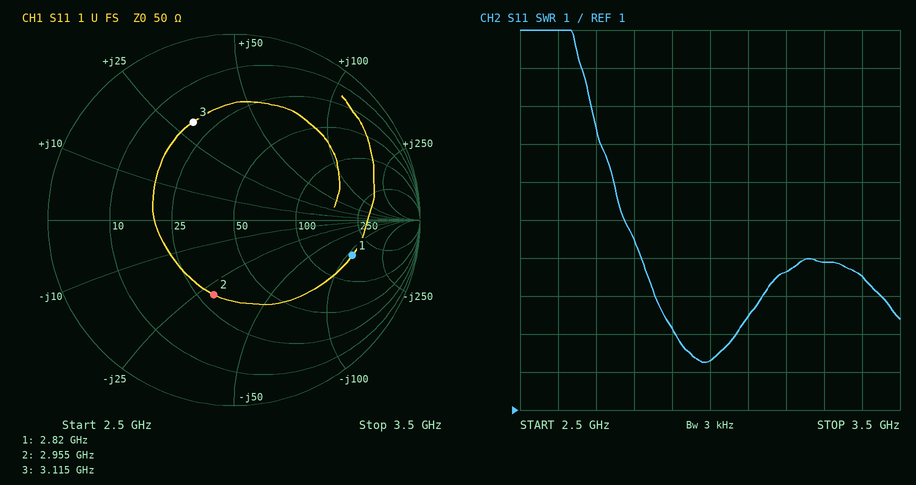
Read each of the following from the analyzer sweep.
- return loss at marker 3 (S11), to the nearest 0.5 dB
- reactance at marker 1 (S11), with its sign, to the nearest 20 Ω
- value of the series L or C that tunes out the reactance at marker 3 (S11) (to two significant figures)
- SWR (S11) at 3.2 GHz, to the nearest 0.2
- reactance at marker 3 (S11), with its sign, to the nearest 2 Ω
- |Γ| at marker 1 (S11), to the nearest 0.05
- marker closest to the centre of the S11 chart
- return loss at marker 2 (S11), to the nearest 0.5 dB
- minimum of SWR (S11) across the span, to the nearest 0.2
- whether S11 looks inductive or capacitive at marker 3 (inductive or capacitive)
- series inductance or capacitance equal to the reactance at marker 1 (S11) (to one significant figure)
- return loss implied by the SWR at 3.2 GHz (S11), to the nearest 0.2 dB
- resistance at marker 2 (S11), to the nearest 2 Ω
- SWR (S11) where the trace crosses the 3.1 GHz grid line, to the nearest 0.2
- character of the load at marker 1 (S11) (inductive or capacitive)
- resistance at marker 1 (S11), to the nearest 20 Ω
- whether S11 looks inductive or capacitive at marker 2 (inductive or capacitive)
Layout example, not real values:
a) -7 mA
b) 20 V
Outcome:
a) 5.0 dB
b) -120 Ω
c) 1.7 pF
d) 4.6
e) +30 Ω
f) 0.65
g) marker 2
h) 7.5 dB
i) 2.2
j) inductive
k) 500 fF
l) 3.8 dB
m) 30 Ω
n) 3.4
o) capacitive
p) 160 Ω
q) capacitive
